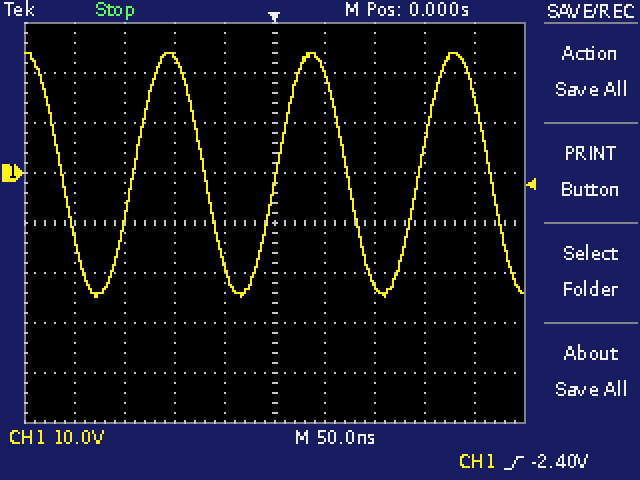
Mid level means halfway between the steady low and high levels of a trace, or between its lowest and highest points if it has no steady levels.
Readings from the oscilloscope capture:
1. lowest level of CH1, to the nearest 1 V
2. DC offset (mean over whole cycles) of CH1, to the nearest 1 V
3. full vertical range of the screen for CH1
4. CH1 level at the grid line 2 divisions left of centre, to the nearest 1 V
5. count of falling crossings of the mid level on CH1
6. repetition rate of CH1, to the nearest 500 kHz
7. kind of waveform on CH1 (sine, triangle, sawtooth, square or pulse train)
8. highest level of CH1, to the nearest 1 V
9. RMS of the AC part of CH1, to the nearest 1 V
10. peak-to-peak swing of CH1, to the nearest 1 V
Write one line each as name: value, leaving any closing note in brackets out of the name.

lowest level of CH1, to the nearest 1 V: -25 V
DC offset (mean over whole cycles) of CH1, to the nearest 1 V: 0 V
full vertical range of the screen for CH1: 80 V
CH1 level at the grid line 2 divisions left of centre, to the nearest 1 V: 23 V
count of falling crossings of the mid level on CH1: 4
repetition rate of CH1, to the nearest 500 kHz: 7.0 MHz
kind of waveform on CH1: sine
highest level of CH1, to the nearest 1 V: 24 V
RMS of the AC part of CH1, to the nearest 1 V: 17 V
peak-to-peak swing of CH1, to the nearest 1 V: 49 V
